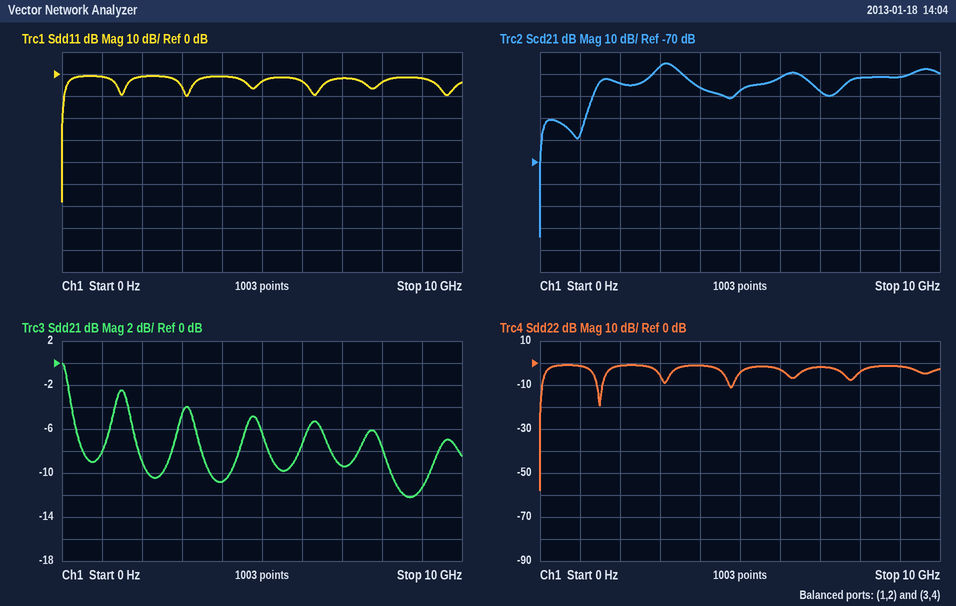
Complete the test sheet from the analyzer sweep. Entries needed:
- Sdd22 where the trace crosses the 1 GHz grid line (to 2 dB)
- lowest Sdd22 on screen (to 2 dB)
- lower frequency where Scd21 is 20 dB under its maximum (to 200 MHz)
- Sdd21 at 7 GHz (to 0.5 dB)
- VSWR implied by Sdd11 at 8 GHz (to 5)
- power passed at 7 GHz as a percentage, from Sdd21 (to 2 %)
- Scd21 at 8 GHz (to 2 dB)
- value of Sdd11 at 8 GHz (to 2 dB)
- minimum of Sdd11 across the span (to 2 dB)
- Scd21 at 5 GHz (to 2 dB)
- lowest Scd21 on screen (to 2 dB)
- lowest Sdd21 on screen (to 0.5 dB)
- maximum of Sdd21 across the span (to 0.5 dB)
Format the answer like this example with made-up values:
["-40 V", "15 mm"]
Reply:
["-2 dB", "-58 dB", "1.2 GHz", "-9.5 dB", "5", "12 %", "-32 dB", "-4 dB", "-58 dB", "-38 dB", "-104 dB", "-12.0 dB", "0.0 dB"]
